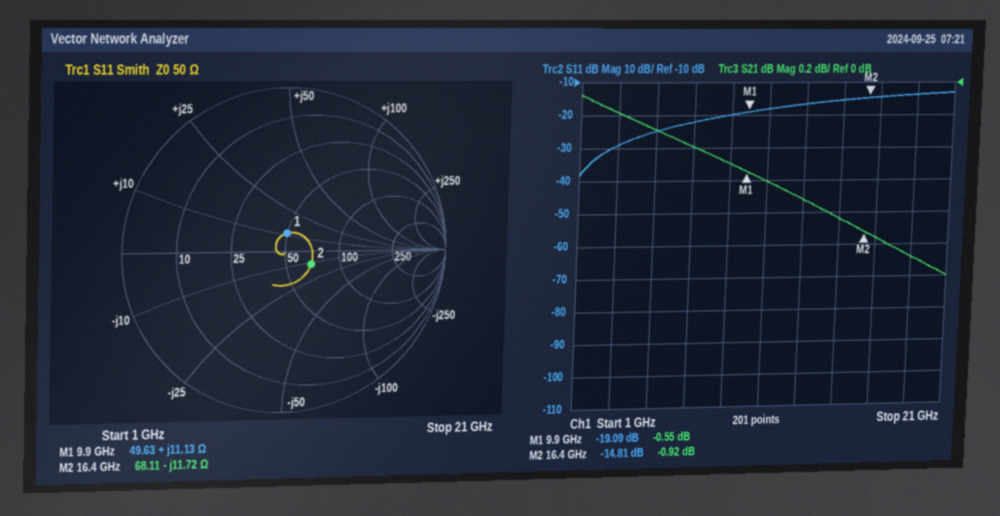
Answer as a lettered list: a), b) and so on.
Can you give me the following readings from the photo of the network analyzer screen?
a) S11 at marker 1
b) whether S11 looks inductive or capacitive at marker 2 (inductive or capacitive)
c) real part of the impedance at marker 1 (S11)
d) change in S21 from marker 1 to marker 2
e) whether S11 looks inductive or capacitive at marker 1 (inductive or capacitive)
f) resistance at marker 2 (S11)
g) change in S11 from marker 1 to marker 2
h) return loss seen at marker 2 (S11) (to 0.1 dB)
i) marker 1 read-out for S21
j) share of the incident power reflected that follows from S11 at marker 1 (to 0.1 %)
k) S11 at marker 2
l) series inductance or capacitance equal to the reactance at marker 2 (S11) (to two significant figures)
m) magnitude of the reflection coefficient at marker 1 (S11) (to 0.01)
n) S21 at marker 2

a) -19.09 dB
b) capacitive
c) 49.63 Ω
d) -0.37 dB
e) inductive
f) 68.11 Ω
g) 4.28 dB
h) 14.8 dB
i) -0.55 dB
j) 1.2 %
k) -14.81 dB
l) 830 fF
m) 0.11
n) -0.92 dB
